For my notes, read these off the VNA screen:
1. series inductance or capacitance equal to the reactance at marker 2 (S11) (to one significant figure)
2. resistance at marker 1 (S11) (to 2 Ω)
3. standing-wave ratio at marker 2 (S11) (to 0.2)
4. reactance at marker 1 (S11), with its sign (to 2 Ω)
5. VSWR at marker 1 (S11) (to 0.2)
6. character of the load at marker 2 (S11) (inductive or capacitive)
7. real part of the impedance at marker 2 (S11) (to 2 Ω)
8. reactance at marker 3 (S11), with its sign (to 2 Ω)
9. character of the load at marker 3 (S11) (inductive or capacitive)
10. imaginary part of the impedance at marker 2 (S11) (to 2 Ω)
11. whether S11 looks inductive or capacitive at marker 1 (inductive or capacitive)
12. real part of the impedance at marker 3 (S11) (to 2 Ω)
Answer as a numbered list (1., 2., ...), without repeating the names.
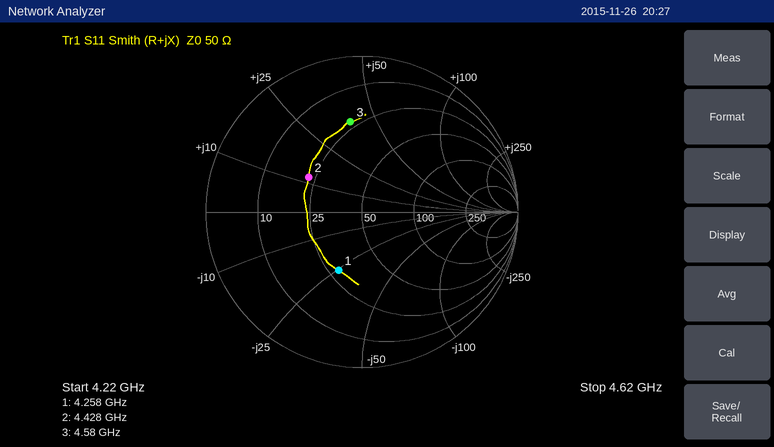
1. 400 pH
2. 28 Ω
3. 2.4
4. -26 Ω
5. 2.4
6. inductive
7. 22 Ω
8. +38 Ω
9. inductive
10. +12 Ω
11. capacitive
12. 22 Ω
